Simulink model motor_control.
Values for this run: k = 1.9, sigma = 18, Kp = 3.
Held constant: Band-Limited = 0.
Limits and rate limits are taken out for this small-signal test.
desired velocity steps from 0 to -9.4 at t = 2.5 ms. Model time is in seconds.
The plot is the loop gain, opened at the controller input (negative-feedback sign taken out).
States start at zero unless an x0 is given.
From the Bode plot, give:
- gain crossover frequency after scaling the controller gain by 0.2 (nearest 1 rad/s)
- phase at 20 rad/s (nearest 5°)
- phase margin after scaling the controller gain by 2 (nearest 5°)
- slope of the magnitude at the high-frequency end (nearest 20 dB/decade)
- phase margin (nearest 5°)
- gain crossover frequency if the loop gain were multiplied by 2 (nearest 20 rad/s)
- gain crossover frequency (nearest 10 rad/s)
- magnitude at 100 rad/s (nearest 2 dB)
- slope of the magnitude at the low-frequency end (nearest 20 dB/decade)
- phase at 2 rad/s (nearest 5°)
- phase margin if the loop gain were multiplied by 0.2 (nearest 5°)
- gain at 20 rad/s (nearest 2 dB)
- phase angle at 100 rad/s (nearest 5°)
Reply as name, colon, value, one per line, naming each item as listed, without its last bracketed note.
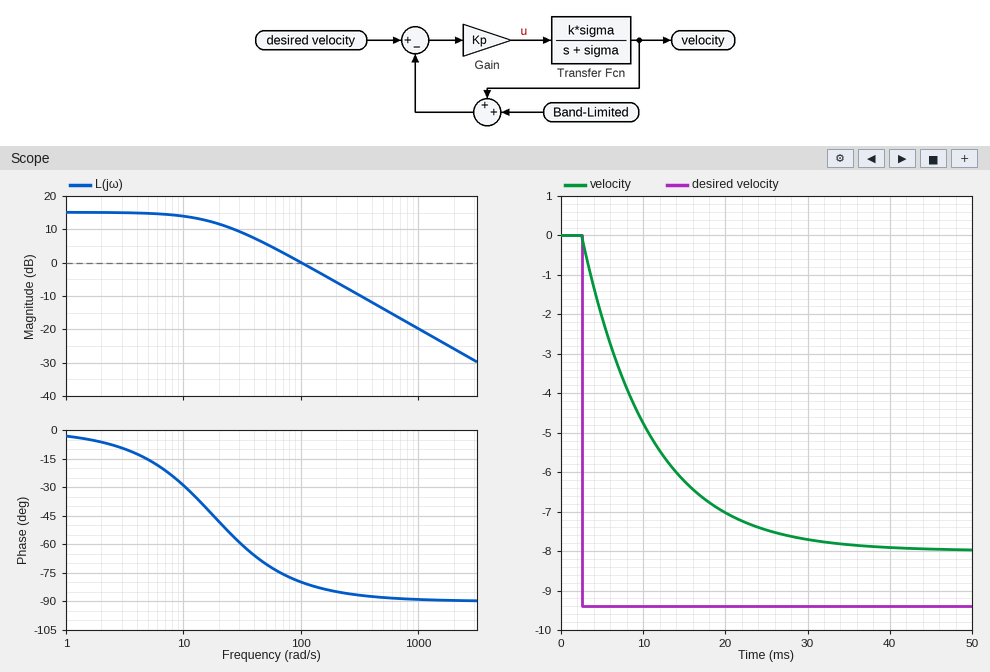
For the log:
gain crossover frequency after scaling the controller gain by 0.2: 10 rad/s
phase at 20 rad/s: -50°
phase margin after scaling the controller gain by 2: 95°
slope of the magnitude at the high-frequency end: -20 dB/decade
phase margin: 100°
gain crossover frequency if the loop gain were multiplied by 2: 200 rad/s
gain crossover frequency: 100 rad/s
magnitude at 100 rad/s: 0 dB
slope of the magnitude at the low-frequency end: 0 dB/decade
phase at 2 rad/s: -5°
phase margin if the loop gain were multiplied by 0.2: 150°
gain at 20 rad/s: 12 dB
phase angle at 100 rad/s: -80°
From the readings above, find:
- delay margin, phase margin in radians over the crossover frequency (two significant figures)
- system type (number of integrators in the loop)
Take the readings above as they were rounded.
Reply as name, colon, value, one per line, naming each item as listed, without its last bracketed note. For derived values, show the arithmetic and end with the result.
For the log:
delay margin, phase margin in radians over the crossover frequency: 100 × π / 180 / 100 = 0.017 s
system type: 0
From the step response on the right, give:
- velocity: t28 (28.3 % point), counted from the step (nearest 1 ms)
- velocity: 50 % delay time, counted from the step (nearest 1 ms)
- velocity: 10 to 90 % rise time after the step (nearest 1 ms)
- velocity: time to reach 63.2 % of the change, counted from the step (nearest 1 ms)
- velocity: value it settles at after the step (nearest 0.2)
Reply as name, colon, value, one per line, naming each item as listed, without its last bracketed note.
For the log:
velocity: t28 (28.3 % point), counted from the step: 3 ms
velocity: 50 % delay time, counted from the step: 6 ms
velocity: 10 to 90 % rise time after the step: 18 ms
velocity: time to reach 63.2 % of the change, counted from the step: 8 ms
velocity: value it settles at after the step: -8.0
